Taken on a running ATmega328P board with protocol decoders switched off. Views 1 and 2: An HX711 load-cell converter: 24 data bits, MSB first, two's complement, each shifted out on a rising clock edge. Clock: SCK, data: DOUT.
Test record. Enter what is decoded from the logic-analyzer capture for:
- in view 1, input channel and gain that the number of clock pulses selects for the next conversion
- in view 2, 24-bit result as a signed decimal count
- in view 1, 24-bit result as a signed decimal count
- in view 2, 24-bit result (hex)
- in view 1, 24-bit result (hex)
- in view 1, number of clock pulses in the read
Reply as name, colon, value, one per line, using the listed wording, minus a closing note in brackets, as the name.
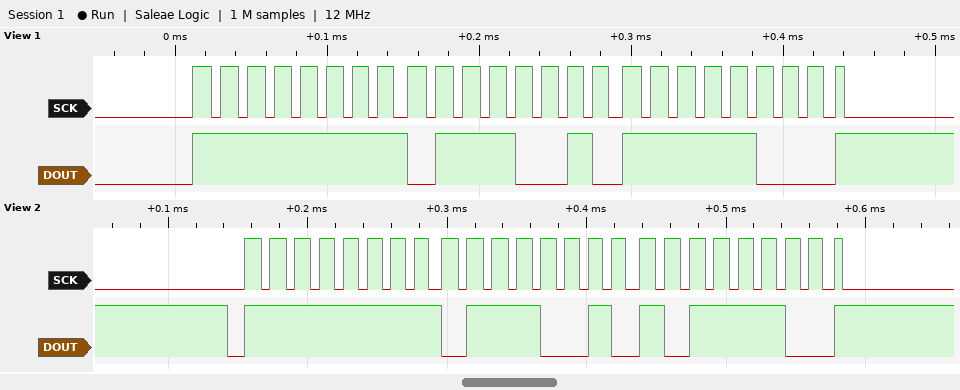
in view 1, input channel and gain that the number of clock pulses selects for the next conversion: channel A, gain 128
in view 2, 24-bit result as a signed decimal count: -36164
in view 1, 24-bit result as a signed decimal count: -36104
in view 2, 24-bit result: 0xFF72BC
in view 1, 24-bit result: 0xFF72F8
in view 1, number of clock pulses in the read: 25
